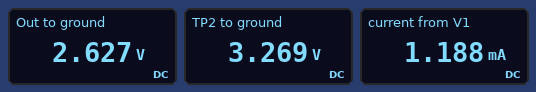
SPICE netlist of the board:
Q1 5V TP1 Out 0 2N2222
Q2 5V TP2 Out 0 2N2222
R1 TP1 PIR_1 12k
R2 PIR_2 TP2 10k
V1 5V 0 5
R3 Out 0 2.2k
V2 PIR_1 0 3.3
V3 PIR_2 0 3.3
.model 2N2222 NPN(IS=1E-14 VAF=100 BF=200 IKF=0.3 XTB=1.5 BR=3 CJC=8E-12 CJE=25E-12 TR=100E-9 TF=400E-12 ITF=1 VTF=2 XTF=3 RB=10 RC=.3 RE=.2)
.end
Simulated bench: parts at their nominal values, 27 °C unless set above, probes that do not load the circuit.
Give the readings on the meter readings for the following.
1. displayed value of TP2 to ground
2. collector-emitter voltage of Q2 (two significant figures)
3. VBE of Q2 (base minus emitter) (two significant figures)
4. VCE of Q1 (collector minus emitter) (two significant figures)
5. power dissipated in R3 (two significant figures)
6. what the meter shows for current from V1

3.269 V
2.4 V
640 mV
2.4 V
3.1 mW
1.188 mA
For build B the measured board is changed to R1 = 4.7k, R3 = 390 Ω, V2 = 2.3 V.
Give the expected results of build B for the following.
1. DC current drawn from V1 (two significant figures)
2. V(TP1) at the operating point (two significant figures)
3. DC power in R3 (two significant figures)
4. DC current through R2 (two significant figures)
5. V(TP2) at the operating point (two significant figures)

5.9 mA
2.3 V
14 mW
29 µA
3.0 V
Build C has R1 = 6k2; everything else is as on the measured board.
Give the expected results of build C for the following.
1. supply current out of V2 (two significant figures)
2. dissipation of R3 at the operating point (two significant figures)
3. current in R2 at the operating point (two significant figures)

3.3 µA
3.2 mW
2.6 µA
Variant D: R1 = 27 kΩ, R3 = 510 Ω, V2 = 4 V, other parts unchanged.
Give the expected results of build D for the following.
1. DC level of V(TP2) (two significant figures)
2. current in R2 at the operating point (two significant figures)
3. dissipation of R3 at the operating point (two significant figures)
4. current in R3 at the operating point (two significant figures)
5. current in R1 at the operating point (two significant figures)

3.3 V
1.8 µA
14 mW
5.2 mA
24 µA
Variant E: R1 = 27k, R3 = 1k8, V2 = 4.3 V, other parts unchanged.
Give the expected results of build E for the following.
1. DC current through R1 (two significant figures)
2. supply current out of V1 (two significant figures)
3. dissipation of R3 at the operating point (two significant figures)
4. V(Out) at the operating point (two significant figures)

9.3 µA
1.9 mA
6.3 mW
3.4 V
